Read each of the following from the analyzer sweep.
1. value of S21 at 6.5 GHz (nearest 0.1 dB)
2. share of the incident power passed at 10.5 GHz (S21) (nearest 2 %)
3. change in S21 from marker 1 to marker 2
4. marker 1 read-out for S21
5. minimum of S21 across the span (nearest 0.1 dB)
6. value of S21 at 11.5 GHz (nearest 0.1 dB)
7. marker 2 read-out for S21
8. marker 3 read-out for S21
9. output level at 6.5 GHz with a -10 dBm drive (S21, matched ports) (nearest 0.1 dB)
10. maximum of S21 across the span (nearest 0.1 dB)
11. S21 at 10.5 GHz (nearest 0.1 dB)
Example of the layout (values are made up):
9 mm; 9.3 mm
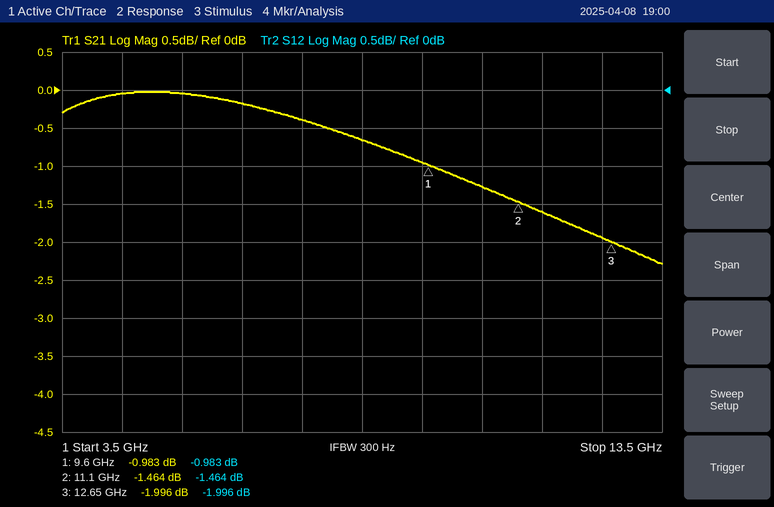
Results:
-0.2 dB; 74 %; -0.481 dB; -0.983 dB; -2.3 dB; -1.6 dB; -1.464 dB; -1.996 dB; -10.2 dBm; 0.0 dB; -1.3 dB
